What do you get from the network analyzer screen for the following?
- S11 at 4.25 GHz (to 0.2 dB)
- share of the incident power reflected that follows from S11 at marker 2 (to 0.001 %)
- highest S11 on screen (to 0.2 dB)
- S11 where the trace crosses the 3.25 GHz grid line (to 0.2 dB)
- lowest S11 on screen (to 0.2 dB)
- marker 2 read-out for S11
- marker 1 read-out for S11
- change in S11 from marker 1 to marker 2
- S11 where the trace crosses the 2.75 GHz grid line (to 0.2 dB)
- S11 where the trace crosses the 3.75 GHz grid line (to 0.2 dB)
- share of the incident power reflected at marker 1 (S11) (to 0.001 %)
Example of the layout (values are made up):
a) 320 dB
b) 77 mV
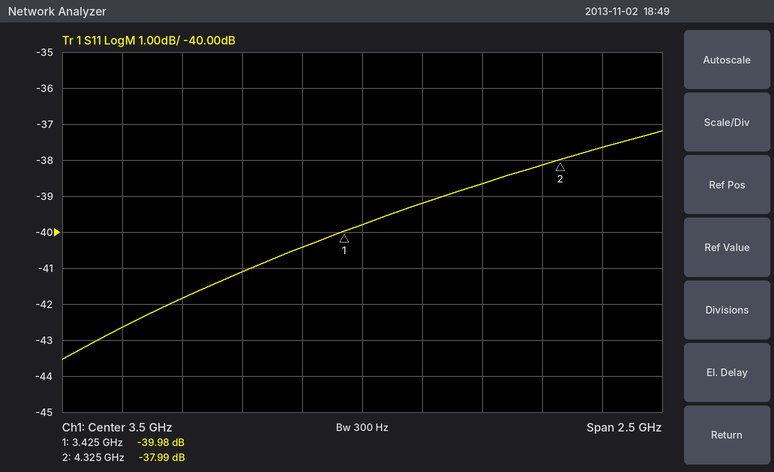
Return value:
a) -38.2 dB
b) 0.016 %
c) -37.2 dB
d) -40.4 dB
e) -43.6 dB
f) -37.99 dB
g) -39.98 dB
h) 1.99 dB
i) -41.8 dB
j) -39.2 dB
k) 0.010 %
